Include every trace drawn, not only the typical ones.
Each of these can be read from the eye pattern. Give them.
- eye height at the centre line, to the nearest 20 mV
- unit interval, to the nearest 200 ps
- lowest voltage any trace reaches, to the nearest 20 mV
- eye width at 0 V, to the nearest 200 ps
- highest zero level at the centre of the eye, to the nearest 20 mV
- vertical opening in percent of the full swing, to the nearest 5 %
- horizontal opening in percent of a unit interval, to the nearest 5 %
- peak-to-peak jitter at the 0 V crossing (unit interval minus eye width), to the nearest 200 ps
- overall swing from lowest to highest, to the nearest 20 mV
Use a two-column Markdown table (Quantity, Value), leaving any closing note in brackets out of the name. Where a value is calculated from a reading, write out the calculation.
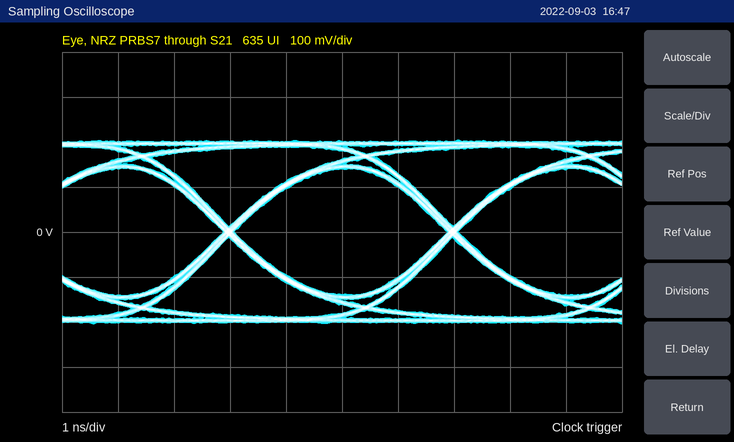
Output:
| Quantity | Value |
|---|---|
| eye height at the centre line, to the nearest 20 mV | 280 mV |
| unit interval, to the nearest 200 ps | 4.0 ns |
| lowest voltage any trace reaches, to the nearest 20 mV | -200 mV |
| eye width at 0 V, to the nearest 200 ps | 3.8 ns |
| highest zero level at the centre of the eye, to the nearest 20 mV | -140 mV |
| vertical opening in percent of the full swing, to the nearest 5 % | 280 mV / 400 mV ≈ 70 % |
| horizontal opening in percent of a unit interval, to the nearest 5 % | 3.8 ns / 4.0 ns ≈ 95 % |
| peak-to-peak jitter at the 0 V crossing (unit interval minus eye width), to the nearest 200 ps | 200 ps |
| overall swing from lowest to highest, to the nearest 20 mV | 400 mV |
